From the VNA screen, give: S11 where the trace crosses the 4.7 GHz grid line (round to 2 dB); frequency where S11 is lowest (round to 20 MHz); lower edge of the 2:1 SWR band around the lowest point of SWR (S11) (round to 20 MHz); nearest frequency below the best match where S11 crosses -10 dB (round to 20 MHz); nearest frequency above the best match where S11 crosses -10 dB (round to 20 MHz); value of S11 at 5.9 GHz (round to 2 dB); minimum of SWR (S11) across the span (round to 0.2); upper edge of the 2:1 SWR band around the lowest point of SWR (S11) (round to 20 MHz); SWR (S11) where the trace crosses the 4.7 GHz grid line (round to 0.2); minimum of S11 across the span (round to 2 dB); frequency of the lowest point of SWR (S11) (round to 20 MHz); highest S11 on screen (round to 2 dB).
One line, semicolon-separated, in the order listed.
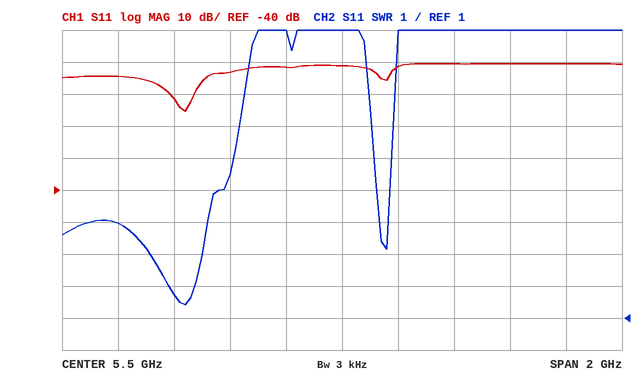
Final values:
-4 dB; 4.94 GHz; 4.88 GHz; 4.88 GHz; 4.98 GHz; 0 dB; 1.4; 4.98 GHz; 4.0; -16 dB; 4.94 GHz; 0 dB
